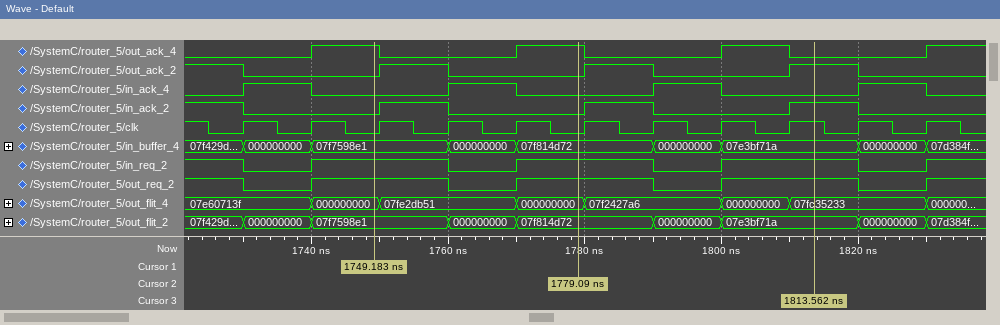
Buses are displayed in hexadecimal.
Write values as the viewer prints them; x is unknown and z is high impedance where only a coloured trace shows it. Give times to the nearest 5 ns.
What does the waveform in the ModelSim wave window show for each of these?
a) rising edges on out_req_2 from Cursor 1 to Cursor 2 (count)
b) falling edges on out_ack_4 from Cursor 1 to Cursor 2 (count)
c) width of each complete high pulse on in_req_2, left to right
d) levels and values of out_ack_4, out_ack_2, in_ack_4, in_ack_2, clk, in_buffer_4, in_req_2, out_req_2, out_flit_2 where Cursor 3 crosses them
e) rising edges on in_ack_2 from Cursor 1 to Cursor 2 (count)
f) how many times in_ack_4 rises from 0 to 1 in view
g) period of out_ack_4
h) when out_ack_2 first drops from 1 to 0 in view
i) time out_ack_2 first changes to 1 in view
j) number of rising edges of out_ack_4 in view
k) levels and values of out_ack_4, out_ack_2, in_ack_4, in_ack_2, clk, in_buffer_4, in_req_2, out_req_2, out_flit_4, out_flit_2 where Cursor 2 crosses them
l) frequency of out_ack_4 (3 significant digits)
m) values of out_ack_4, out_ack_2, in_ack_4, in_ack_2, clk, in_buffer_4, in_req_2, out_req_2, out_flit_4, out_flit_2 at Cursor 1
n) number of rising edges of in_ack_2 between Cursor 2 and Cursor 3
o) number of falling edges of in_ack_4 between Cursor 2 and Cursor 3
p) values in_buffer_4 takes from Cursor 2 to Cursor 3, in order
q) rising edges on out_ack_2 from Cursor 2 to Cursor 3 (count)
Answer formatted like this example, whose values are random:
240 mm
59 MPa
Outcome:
1
1
20 ns, 20 ns, 20 ns
out_ack_4=0, out_ack_2=1, in_ack_4=0, in_ack_2=1, clk=1, in_buffer_4=07e3bf71a, in_req_2=1, out_req_2=1, out_flit_2=07e3bf71a
1
4
30 ns
1730 ns
1750 ns
4
out_ack_4=1, out_ack_2=0, in_ack_4=0, in_ack_2=0, clk=0, in_buffer_4=07f814d72, in_req_2=1, out_req_2=1, out_flit_4=000000000, out_flit_2=07f814d72
33.3 MHz
out_ack_4=1, out_ack_2=0, in_ack_4=0, in_ack_2=0, clk=0, in_buffer_4=07f7598e1, in_req_2=1, out_req_2=1, out_flit_4=000000000, out_flit_2=07f7598e1
2
1
07f814d72, 000000000, 07e3bf71a
2
